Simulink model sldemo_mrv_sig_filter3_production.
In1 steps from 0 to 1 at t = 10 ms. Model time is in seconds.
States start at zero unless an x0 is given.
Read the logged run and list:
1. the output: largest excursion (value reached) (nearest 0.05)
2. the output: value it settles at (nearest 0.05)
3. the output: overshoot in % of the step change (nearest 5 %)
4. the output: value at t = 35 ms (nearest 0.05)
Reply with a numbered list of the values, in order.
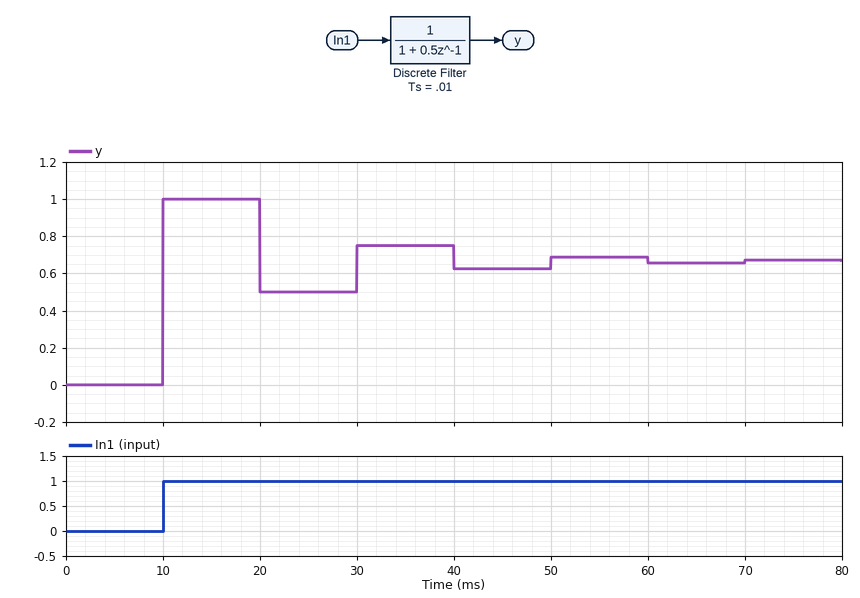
1. 1.00
2. 0.65
3. 50 %
4. 0.75
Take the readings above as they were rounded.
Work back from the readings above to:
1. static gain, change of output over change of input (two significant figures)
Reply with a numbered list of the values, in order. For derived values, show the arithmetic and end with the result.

1. (0.65 - 0) / (1 - 0) = 0.65
